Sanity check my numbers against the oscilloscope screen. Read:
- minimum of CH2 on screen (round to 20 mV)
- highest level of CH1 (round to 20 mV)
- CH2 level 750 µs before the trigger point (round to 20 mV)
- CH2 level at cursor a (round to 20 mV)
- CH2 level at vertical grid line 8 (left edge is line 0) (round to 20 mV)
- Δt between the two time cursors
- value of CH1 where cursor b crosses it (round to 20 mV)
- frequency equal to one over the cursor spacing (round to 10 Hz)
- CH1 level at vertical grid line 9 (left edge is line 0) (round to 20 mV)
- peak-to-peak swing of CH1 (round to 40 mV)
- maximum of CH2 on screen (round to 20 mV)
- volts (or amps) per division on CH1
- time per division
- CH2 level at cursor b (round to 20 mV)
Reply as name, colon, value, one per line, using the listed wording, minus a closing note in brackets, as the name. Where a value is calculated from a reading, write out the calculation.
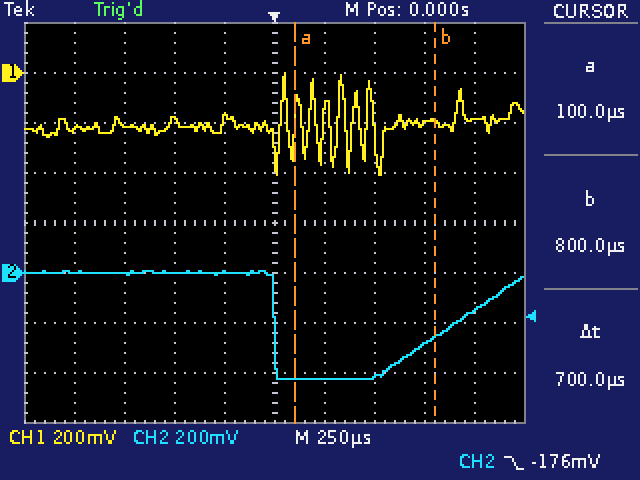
minimum of CH2 on screen: -420 mV
highest level of CH1: 0 mV
CH2 level 750 µs before the trigger point: 0 mV
CH2 level at cursor a: -420 mV
CH2 level at vertical grid line 8 (left edge is line 0): -280 mV
Δt between the two time cursors: 700 µs
value of CH1 where cursor b crosses it: -200 mV
frequency equal to one over the cursor spacing: 1 / 700 µs ≈ 1.43 kHz
CH1 level at vertical grid line 9 (left edge is line 0): -180 mV
peak-to-peak swing of CH1: 400 mV
maximum of CH2 on screen: 0 mV
volts (or amps) per division on CH1: 200 mV
time per division: 250 µs
CH2 level at cursor b: -260 mV
